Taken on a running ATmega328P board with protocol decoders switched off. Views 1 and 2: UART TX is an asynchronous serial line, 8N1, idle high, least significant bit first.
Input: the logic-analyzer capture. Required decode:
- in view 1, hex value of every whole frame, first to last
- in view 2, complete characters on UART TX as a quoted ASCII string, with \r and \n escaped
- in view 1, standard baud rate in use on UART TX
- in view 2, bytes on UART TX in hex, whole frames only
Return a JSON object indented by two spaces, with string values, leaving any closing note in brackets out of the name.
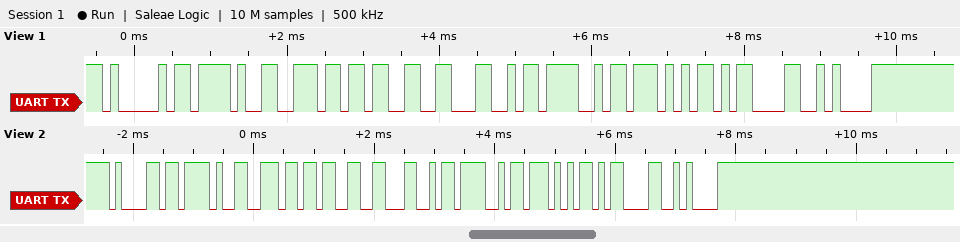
{
  "in view 1, hex value of every whole frame, first to last": "41 2F 6E 33 4C 4F 57 0D 0A",
  "in view 2, complete characters on UART TX as a quoted ASCII string, with \\r and \\n escaped": "\"a/n3LOW\\r\\n\"",
  "in view 1, standard baud rate in use on UART TX": "9600 baud",
  "in view 2, bytes on UART TX in hex, whole frames only": "61 2F 6E 33 4C 4F 57 0D 0A"
}
